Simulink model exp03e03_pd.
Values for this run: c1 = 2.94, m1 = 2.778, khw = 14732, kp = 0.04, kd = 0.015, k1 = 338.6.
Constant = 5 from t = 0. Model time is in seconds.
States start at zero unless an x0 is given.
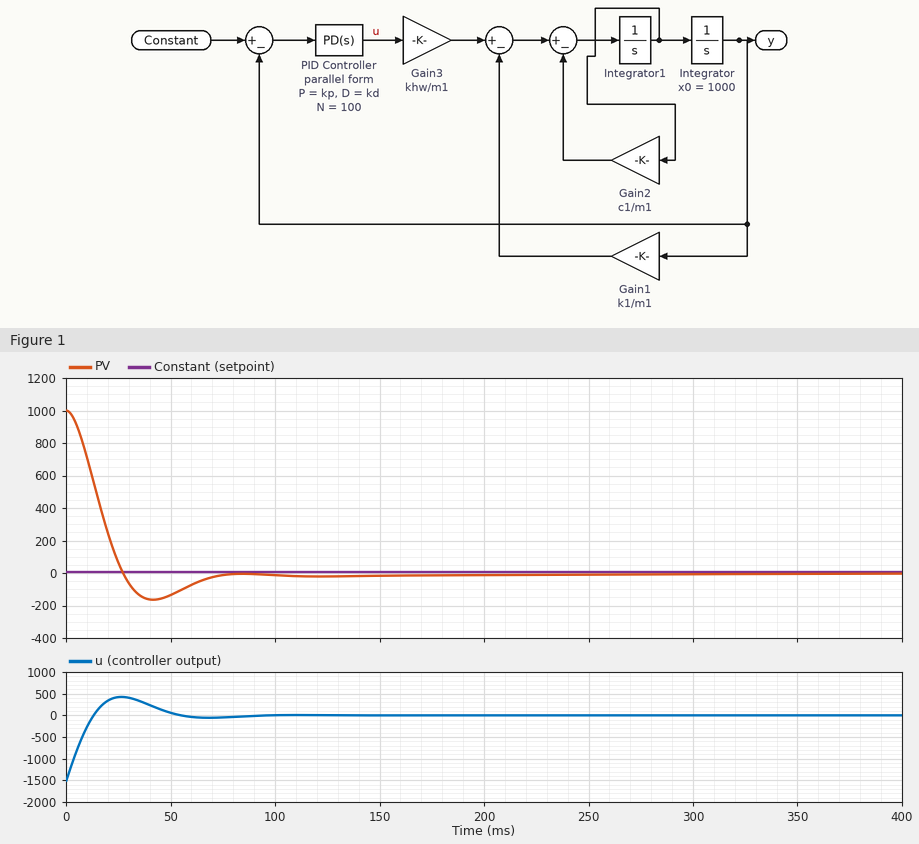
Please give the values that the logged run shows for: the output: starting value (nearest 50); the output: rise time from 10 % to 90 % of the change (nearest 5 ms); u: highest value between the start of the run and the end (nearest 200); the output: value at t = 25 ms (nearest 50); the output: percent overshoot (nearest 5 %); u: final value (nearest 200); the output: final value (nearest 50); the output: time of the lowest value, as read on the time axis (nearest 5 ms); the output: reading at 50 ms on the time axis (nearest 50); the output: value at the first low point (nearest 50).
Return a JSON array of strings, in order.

["1000", "20 ms", "400", "50", "15 %", "0", "0", "40 ms", "-150", "-150"]
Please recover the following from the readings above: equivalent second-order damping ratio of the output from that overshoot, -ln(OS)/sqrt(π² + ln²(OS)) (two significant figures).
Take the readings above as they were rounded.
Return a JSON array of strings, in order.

["0.52"]
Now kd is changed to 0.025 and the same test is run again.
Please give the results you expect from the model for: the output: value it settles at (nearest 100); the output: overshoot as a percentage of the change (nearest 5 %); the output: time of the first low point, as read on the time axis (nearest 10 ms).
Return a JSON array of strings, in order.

["0", "25 %", "30 ms"]
